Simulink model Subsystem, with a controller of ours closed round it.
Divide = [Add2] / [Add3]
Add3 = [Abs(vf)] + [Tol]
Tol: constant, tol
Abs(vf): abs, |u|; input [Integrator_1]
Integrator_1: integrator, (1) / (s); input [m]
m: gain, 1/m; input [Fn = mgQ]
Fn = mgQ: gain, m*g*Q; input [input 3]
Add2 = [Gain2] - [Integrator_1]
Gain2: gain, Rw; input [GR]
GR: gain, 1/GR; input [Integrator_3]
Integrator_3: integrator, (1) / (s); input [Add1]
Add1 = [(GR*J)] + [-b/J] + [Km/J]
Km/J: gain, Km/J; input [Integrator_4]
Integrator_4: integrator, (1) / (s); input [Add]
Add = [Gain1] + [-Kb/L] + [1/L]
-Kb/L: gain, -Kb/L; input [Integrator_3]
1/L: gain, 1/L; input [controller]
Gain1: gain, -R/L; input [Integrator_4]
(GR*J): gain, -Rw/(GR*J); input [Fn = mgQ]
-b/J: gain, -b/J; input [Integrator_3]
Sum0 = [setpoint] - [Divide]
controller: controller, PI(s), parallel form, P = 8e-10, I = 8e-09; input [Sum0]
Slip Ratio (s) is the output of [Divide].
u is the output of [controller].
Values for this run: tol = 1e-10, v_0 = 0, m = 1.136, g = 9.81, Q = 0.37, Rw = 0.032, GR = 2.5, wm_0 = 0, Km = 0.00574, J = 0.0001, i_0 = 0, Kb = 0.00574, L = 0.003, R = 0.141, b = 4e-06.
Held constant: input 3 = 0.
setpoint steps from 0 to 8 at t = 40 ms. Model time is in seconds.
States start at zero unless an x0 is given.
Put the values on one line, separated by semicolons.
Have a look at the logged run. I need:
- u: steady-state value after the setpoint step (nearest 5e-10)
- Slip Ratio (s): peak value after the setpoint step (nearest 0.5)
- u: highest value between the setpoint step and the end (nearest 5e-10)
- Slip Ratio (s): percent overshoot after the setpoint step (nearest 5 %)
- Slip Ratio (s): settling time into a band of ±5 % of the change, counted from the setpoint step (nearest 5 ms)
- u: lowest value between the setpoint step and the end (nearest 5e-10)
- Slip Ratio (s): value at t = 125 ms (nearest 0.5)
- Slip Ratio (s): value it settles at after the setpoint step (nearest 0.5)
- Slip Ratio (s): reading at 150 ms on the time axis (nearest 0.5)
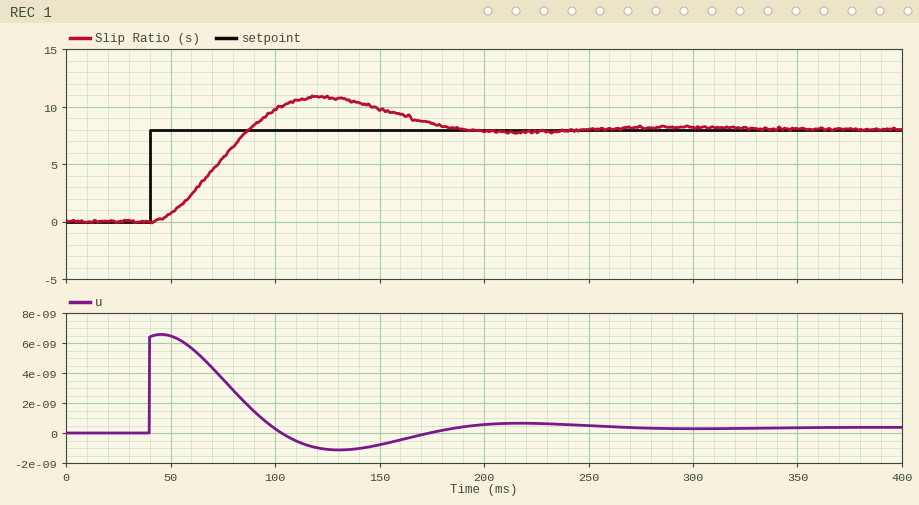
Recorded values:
0.0000000005; 11.0; 0.0000000065; 35 %; 140 ms; -0.0000000010; 11.0; 8.0; 10.0
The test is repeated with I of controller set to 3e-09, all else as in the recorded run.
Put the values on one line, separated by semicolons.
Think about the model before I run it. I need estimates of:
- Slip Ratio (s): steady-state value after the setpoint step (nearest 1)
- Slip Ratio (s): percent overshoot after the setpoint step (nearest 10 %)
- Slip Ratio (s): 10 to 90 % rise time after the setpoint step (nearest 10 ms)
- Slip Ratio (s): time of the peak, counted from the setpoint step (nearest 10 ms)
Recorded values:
8; 20 %; 40 ms; 80 ms
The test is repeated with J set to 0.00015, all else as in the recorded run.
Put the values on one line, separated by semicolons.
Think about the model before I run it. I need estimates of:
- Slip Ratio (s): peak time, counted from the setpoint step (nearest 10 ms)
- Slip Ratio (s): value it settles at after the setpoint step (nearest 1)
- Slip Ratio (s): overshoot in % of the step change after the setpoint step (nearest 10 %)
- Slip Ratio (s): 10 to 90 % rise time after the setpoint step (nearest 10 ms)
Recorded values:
110 ms; 8; 30 %; 40 ms
